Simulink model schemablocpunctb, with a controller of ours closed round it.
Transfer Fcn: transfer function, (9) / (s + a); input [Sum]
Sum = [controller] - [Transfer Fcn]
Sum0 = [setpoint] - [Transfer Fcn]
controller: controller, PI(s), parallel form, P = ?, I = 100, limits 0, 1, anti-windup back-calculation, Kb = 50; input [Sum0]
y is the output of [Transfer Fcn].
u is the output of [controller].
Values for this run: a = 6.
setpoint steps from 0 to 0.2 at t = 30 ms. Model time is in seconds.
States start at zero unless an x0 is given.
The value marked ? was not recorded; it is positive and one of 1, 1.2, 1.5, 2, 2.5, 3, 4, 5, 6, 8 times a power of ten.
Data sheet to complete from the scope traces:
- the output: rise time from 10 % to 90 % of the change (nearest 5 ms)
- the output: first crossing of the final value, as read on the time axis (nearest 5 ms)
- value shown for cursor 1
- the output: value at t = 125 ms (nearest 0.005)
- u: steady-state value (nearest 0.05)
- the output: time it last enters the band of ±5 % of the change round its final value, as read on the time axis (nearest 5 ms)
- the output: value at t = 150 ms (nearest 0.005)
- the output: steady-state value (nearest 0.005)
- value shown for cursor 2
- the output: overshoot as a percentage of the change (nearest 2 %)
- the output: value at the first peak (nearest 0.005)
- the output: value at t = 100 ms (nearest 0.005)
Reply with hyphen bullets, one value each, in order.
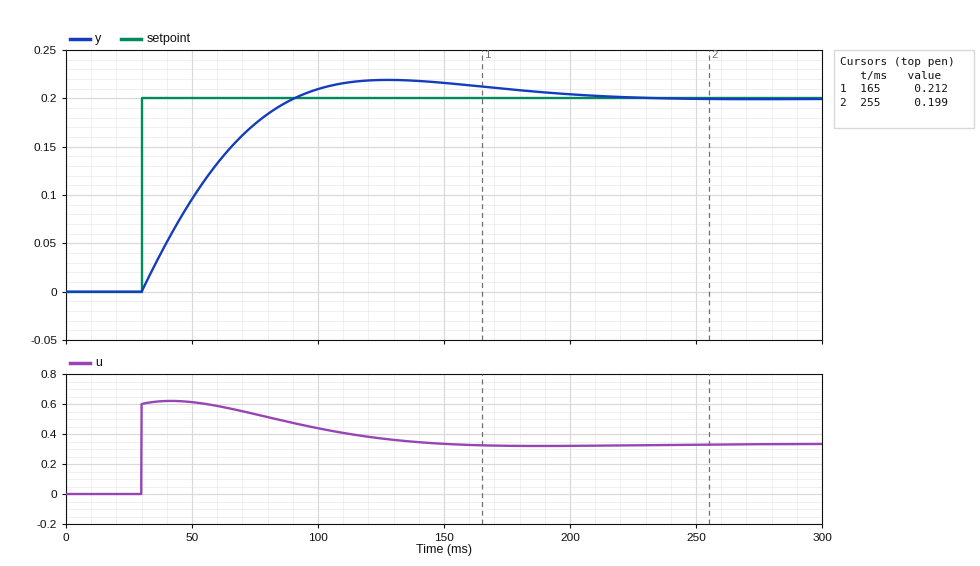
- 45 ms
- 90 ms
- 0.212
- 0.220
- 0.35
- 175 ms
- 0.215
- 0.200
- 0.199
- 10 %
- 0.220
- 0.210
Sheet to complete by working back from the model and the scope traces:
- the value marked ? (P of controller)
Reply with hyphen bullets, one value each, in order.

- 3
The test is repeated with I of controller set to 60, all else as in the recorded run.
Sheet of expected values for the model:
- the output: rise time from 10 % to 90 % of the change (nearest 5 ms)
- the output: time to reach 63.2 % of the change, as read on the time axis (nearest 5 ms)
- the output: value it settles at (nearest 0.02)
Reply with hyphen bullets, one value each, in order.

- 65 ms
- 65 ms
- 0.20
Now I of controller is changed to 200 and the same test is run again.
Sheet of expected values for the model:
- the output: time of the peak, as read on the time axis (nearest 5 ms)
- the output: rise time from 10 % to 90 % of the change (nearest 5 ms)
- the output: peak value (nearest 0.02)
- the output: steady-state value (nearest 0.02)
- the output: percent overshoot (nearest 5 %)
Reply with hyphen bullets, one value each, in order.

- 95 ms
- 30 ms
- 0.24
- 0.20
- 20 %
